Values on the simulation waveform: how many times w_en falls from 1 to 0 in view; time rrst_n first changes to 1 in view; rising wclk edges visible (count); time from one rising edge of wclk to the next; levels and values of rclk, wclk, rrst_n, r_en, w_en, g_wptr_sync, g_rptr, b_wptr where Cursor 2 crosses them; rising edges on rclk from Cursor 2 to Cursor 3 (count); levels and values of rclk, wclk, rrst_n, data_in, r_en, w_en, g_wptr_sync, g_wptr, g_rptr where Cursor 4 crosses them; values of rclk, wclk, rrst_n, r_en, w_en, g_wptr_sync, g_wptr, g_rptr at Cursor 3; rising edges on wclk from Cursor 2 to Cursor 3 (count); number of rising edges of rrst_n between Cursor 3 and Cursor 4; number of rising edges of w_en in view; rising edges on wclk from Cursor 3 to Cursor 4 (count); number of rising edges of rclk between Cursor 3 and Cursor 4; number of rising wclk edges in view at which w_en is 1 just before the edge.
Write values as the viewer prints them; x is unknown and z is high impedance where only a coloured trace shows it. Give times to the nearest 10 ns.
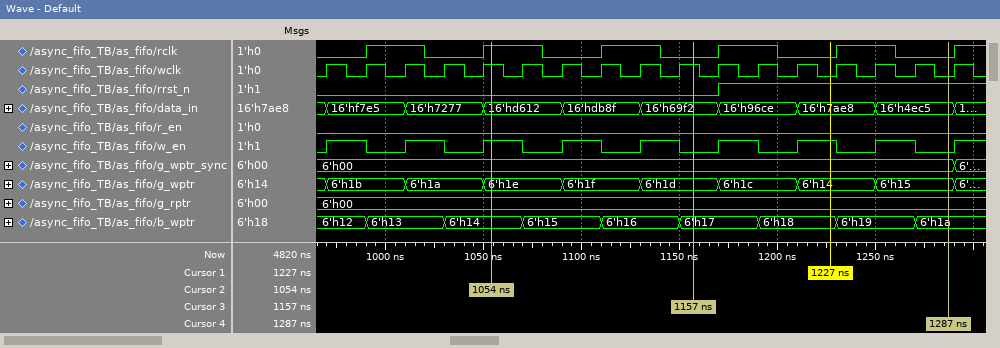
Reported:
8
1170 ns
17
20 ns
rclk=1, wclk=1, rrst_n=0, r_en=0, w_en=1, g_wptr_sync=6'h00, g_rptr=6'h00, b_wptr=6'h14
1
rclk=0, wclk=0, rrst_n=1, data_in=16'h4ec5, r_en=0, w_en=0, g_wptr_sync=6'h00, g_wptr=6'h15, g_rptr=6'h00
rclk=0, wclk=1, rrst_n=0, r_en=0, w_en=0, g_wptr_sync=6'h00, g_wptr=6'h1d, g_rptr=6'h00
5
1
9
6
2
8
